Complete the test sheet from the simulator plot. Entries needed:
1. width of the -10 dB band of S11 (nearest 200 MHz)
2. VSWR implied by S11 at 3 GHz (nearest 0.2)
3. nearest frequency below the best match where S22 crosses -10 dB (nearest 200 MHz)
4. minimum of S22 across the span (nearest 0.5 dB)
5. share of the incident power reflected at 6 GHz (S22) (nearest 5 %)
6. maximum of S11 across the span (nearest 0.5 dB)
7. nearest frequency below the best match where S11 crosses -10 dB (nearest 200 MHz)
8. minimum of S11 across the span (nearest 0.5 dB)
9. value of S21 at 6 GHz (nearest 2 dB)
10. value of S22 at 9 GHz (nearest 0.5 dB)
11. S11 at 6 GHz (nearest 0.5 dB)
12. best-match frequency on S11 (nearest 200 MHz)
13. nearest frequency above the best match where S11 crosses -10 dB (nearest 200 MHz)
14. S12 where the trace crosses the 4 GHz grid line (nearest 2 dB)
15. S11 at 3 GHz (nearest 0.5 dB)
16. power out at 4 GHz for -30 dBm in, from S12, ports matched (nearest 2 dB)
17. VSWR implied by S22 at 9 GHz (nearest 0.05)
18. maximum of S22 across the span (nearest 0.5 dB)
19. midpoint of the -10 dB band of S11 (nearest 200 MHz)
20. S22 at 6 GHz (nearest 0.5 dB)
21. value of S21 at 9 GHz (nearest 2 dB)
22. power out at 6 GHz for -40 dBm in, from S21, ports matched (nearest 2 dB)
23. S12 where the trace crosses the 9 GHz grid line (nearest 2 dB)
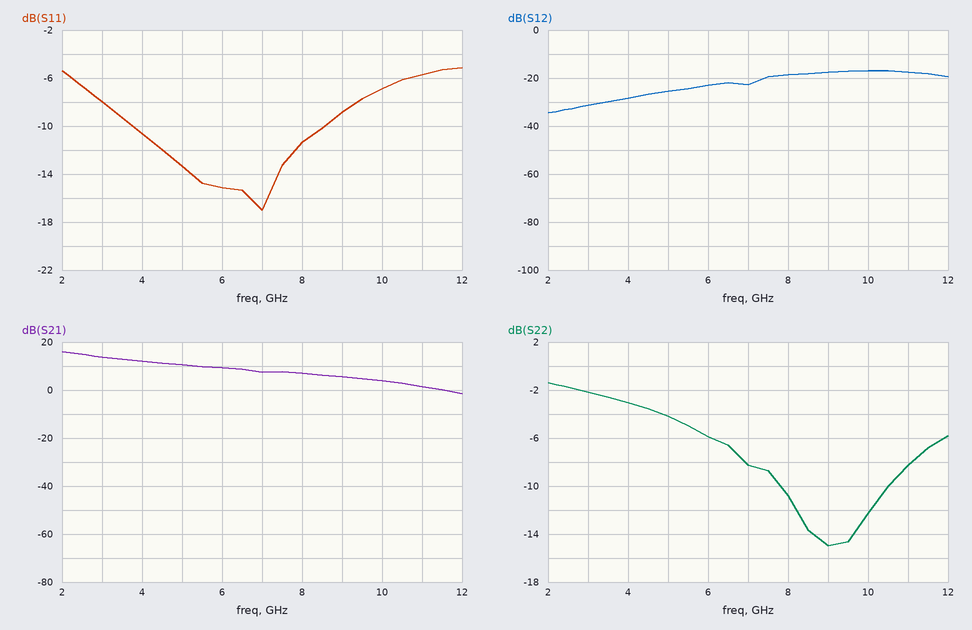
4.8 GHz
2.4
7.8 GHz
-15.0 dB
25 %
-5.0 dB
3.8 GHz
-17.0 dB
10 dB
-15.0 dB
-15.0 dB
7.0 GHz
8.6 GHz
-28 dB
-8.0 dB
-58 dBm
1.45
-1.5 dB
6.2 GHz
-6.0 dB
6 dB
-30 dBm
-18 dB
